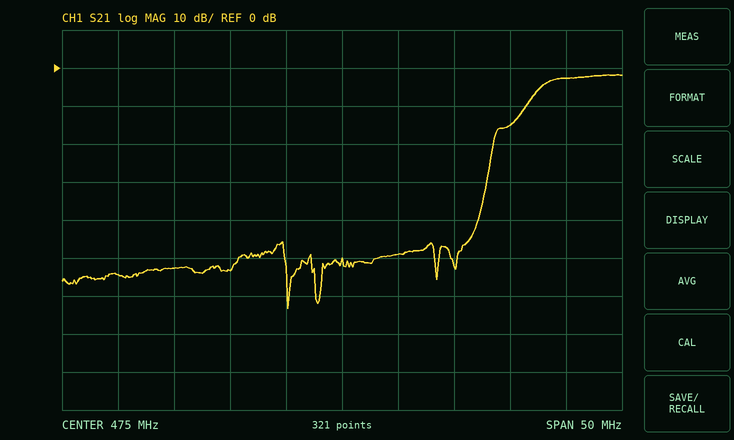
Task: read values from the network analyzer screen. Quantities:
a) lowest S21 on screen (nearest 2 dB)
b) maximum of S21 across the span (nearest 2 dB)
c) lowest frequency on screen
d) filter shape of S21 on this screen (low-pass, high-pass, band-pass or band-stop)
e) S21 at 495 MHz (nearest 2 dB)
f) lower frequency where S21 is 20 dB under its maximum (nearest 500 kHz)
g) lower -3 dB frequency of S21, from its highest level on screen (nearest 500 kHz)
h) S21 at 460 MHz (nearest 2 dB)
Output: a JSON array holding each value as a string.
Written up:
["-64 dB", "-2 dB", "450 MHz", "high-pass", "-2 dB", "488.5 MHz", "493.0 MHz", "-52 dB"]
